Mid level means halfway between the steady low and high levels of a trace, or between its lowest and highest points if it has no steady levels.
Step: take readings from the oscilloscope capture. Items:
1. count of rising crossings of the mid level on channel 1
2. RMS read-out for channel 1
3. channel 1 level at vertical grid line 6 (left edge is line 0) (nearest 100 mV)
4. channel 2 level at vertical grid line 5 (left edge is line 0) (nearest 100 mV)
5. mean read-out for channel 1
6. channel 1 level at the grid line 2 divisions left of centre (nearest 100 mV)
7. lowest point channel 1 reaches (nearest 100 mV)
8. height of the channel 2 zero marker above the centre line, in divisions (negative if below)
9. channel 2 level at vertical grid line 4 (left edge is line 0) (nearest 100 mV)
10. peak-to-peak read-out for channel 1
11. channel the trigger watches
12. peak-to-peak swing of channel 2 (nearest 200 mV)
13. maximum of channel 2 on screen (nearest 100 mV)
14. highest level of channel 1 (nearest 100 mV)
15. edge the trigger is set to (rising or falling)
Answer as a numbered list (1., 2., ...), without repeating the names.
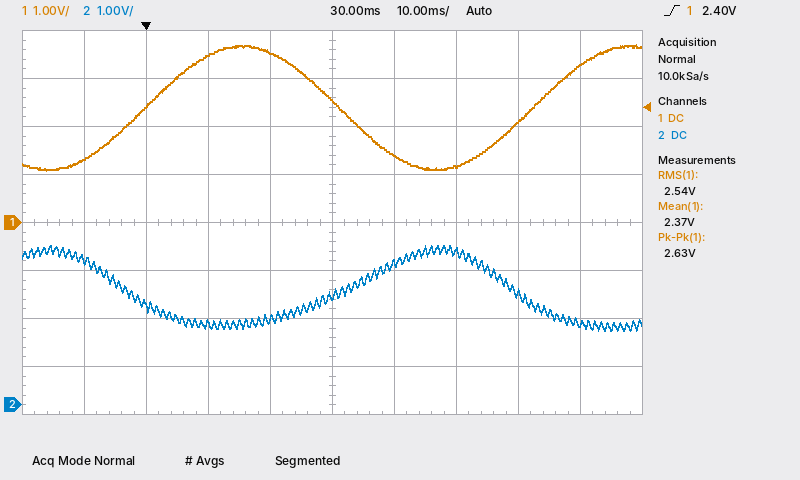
1. 2
2. 2.54 V
3. 1.4 V
4. 2.3 V
5. 2.37 V
6. 3.5 V
7. 1.1 V
8. -3.8 div
9. 1.8 V
10. 2.63 V
11. channel 1
12. 1.8 V
13. 3.3 V
14. 3.7 V
15. rising
